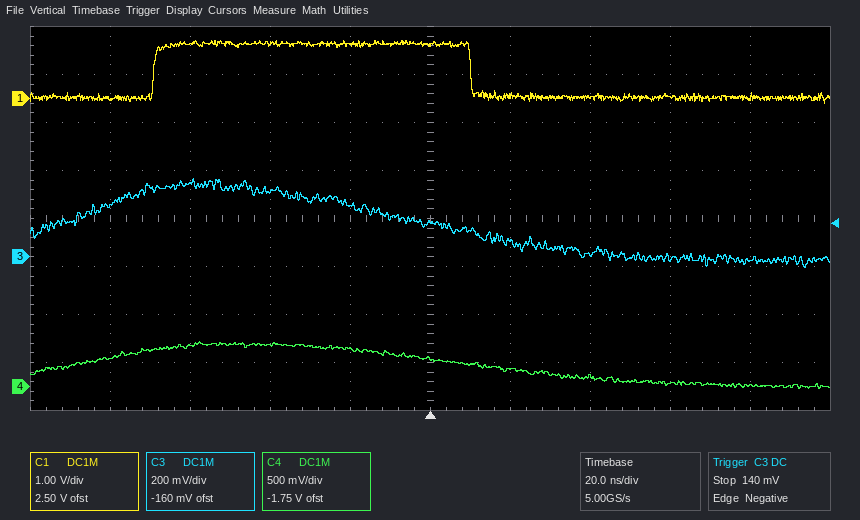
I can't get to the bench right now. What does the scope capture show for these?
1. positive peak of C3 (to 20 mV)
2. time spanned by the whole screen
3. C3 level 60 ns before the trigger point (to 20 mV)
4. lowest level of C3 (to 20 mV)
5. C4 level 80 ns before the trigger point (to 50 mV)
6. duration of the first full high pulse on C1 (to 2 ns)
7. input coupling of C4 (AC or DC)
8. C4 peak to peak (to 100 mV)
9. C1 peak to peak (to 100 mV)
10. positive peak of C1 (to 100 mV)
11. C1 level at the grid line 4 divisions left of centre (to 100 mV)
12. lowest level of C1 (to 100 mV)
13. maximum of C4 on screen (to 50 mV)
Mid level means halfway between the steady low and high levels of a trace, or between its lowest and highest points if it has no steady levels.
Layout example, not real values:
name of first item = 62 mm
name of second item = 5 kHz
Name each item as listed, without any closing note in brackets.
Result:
positive peak of C3 = 320 mV
time spanned by the whole screen = 200 ns
C3 level 60 ns before the trigger point = 320 mV
lowest level of C3 = -40 mV
C4 level 80 ns before the trigger point = 300 mV
duration of the first full high pulse on C1 = 80 ns
input coupling of C4 = DC
C4 peak to peak = 500 mV
C1 peak to peak = 1.3 V
positive peak of C1 = 1.2 V
C1 level at the grid line 4 divisions left of centre = 0.0 V
lowest level of C1 = -100 mV
maximum of C4 on screen = 450 mV
